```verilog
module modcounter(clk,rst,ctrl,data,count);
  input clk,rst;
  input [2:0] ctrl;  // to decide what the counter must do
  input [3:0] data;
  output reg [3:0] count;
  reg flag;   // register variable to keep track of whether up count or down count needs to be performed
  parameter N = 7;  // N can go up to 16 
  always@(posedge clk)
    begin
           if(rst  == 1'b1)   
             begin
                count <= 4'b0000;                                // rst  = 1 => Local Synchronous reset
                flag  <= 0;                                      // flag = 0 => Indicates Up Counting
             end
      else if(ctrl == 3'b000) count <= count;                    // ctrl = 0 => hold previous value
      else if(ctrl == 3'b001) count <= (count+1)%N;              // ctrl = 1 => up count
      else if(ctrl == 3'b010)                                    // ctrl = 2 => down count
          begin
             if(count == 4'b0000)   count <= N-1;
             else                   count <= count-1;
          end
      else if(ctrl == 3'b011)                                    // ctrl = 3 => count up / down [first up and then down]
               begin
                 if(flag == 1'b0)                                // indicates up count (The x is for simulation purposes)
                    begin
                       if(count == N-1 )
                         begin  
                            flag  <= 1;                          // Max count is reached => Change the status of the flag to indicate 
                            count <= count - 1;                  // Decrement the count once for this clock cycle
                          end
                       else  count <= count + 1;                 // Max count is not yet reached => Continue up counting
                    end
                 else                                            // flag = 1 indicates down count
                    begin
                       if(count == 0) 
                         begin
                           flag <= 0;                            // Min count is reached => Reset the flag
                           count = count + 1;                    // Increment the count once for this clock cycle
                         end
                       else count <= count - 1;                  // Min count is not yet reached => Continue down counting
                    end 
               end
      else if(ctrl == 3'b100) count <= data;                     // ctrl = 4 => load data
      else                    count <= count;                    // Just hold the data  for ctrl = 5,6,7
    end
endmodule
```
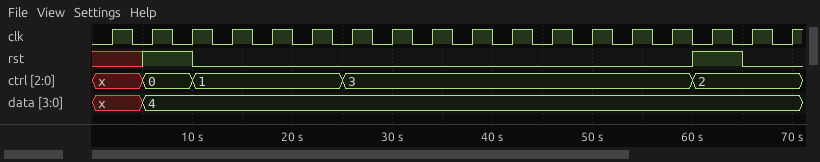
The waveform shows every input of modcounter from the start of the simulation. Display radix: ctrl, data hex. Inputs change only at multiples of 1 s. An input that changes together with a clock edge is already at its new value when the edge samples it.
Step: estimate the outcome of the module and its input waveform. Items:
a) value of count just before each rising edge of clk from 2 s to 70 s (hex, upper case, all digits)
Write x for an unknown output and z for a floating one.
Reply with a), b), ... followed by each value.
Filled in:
a) x, x, 0, 1, 2, 3, 4, 5, 6, 5, 4, 3, 2, 1, 0, 1, 0, 6
